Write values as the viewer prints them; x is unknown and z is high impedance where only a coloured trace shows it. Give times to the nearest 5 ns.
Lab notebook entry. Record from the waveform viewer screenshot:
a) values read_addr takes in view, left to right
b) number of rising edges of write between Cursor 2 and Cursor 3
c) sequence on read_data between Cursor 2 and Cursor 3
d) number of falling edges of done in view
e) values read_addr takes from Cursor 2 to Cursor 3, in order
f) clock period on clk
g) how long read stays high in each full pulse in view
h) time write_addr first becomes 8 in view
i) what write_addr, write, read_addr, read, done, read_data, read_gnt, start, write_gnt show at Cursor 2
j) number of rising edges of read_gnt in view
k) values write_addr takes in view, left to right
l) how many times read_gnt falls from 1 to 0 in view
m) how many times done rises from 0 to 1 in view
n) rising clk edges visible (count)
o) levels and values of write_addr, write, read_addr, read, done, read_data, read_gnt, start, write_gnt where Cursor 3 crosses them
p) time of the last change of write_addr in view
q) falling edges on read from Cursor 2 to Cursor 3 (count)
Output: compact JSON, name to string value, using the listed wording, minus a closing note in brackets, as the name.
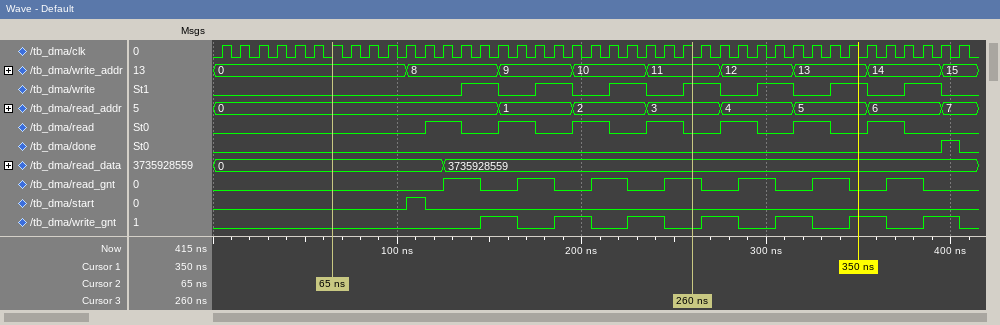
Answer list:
{"values read_addr takes in view, left to right": "0, 1, 2, 3, 4, 5, 6, 7", "number of rising edges of write between Cursor 2 and Cursor 3": "4", "sequence on read_data between Cursor 2 and Cursor 3": "0, 3735928559", "number of falling edges of done in view": "1", "values read_addr takes from Cursor 2 to Cursor 3, in order": "0, 1, 2, 3", "clock period on clk": "10 ns", "how long read stays high in each full pulse in view": "20 ns, 20 ns, 20 ns, 20 ns, 20 ns, 20 ns, 20 ns", "time write_addr first becomes 8 in view": "105 ns", "what write_addr, write, read_addr, read, done, read_data, read_gnt, start, write_gnt show at Cursor 2": "write_addr=0, write=0, read_addr=0, read=0, done=0, read_data=0, read_gnt=0, start=0, write_gnt=0", "number of rising edges of read_gnt in view": "7", "values write_addr takes in view, left to right": "0, 8, 9, 10, 11, 12, 13, 14, 15", "how many times read_gnt falls from 1 to 0 in view": "7", "how many times done rises from 0 to 1 in view": "1", "rising clk edges visible": "41", "levels and values of write_addr, write, read_addr, read, done, read_data, read_gnt, start, write_gnt where Cursor 3 crosses them": "write_addr=11, write=1, read_addr=3, read=0, done=0, read_data=3735928559, read_gnt=1, start=0, write_gnt=0", "time of the last change of write_addr in view": "395 ns", "falling edges on read from Cursor 2 to Cursor 3": "4"}
